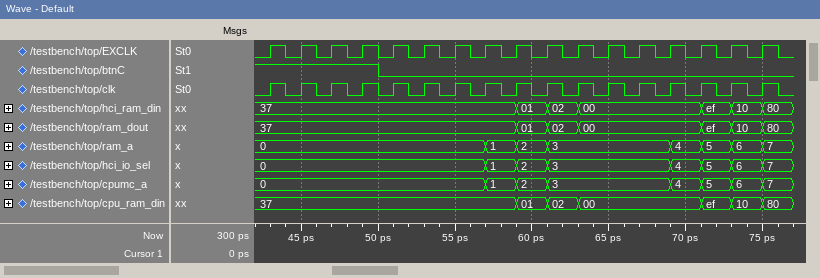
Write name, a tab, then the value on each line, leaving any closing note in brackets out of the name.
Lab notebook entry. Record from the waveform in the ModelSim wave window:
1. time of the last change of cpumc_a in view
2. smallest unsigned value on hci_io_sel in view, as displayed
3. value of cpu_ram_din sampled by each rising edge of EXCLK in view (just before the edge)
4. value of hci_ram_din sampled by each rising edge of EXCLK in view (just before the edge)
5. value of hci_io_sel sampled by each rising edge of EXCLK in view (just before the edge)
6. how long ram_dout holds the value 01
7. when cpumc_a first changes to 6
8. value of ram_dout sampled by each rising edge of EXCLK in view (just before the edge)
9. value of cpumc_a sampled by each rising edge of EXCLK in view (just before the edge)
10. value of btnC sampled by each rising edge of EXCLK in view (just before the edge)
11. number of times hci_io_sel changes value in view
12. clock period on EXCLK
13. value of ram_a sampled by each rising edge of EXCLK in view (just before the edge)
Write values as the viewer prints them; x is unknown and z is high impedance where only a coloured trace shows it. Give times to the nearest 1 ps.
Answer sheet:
time of the last change of cpumc_a in view	75 ps
smallest unsigned value on hci_io_sel in view, as displayed	0
value of cpu_ram_din sampled by each rising edge of EXCLK in view	37, 37, 37, 37, 37, 37, 37, 37, 37, 01, 02, 00, 00, 00, 00, ef, 10
value of hci_ram_din sampled by each rising edge of EXCLK in view	37, 37, 37, 37, 37, 37, 37, 37, 37, 01, 02, 00, 00, 00, 00, ef, 10
value of hci_io_sel sampled by each rising edge of EXCLK in view	0, 0, 0, 0, 0, 0, 0, 0, 1, 2, 3, 3, 3, 3, 4, 5, 6
how long ram_dout holds the value 01	2 ps
when cpumc_a first changes to 6	73 ps
value of ram_dout sampled by each rising edge of EXCLK in view	37, 37, 37, 37, 37, 37, 37, 37, 37, 01, 02, 00, 00, 00, 00, ef, 10
value of cpumc_a sampled by each rising edge of EXCLK in view	0, 0, 0, 0, 0, 0, 0, 0, 1, 2, 3, 3, 3, 3, 4, 5, 6
value of btnC sampled by each rising edge of EXCLK in view	1 1 1 1 0 0 0 0 0 0 0 0 0 0 0 0 0
number of times hci_io_sel changes value in view	7
clock period on EXCLK	2 ps
value of ram_a sampled by each rising edge of EXCLK in view	0, 0, 0, 0, 0, 0, 0, 0, 1, 2, 3, 3, 3, 3, 4, 5, 6
